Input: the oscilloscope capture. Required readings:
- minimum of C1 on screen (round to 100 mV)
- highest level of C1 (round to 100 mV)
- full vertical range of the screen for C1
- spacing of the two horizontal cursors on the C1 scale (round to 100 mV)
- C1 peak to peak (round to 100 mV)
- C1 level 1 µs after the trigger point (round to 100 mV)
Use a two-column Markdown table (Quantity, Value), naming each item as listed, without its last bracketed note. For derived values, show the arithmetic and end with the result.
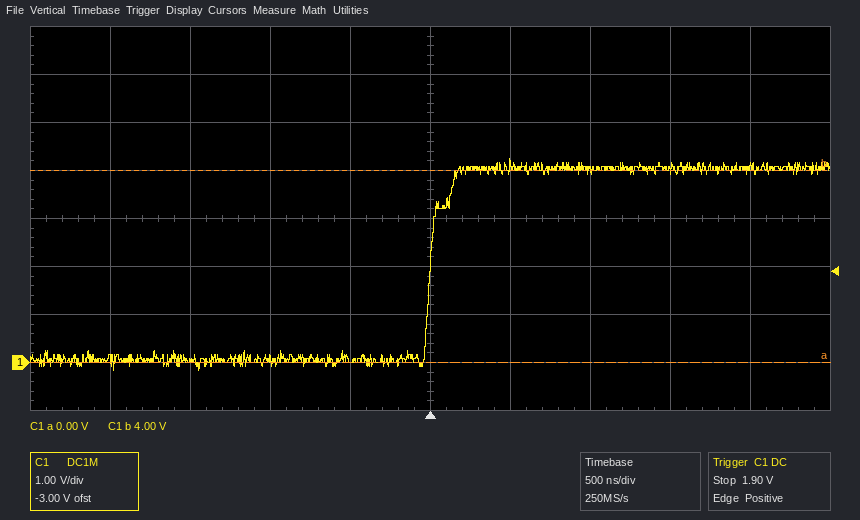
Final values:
| Quantity | Value |
|---|---|
| minimum of C1 on screen | -200 mV |
| highest level of C1 | 4.2 V |
| full vertical range of the screen for C1 | 8 V |
| spacing of the two horizontal cursors on the C1 scale | 4.0 V |
| C1 peak to peak | 4.2 V − (-200 mV) = 4.4 V |
| C1 level 1 µs after the trigger point | 4.0 V |
